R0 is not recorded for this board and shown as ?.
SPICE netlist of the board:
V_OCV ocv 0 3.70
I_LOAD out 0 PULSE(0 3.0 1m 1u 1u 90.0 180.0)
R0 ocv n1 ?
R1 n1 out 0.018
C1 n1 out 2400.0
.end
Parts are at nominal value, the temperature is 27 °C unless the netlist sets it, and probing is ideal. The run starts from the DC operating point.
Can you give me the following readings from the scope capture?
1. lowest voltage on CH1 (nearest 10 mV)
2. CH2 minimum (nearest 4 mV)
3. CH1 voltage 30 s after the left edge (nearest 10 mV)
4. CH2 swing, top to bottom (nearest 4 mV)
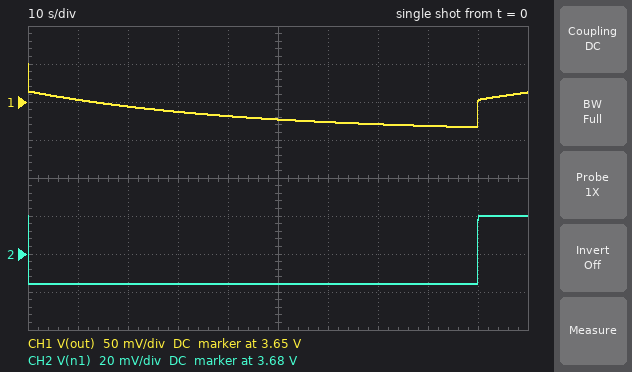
3.62 V
3.664 V
3.64 V
36 mV
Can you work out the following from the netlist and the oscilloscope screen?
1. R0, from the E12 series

0.012 Ω
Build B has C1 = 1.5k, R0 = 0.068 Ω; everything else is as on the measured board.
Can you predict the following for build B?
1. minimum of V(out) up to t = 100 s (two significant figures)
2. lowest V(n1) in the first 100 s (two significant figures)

3.4 V
3.5 V
